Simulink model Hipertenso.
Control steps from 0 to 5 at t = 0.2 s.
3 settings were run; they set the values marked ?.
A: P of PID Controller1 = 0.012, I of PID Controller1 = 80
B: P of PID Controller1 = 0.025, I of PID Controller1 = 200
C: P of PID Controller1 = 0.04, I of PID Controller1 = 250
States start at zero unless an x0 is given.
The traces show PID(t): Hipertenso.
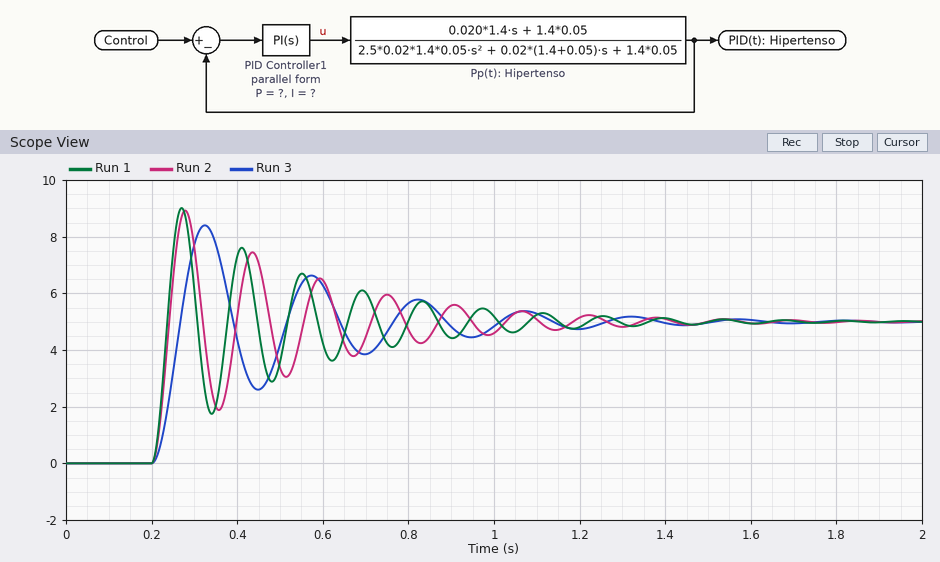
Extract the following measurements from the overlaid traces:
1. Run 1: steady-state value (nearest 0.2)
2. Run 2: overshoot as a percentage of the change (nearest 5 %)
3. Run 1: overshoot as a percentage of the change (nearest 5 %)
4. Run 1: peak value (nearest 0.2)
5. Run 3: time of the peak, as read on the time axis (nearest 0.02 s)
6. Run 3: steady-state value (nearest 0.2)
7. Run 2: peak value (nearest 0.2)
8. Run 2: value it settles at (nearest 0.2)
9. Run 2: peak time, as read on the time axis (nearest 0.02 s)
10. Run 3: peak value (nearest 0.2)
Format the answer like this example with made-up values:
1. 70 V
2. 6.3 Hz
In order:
1. 5.0
2. 80 %
3. 80 %
4. 9.0
5. 0.32 s
6. 5.0
7. 9.0
8. 5.0
9. 0.28 s
10. 8.4
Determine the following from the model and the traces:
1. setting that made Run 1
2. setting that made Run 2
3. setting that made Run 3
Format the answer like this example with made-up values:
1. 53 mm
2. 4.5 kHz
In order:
1. C
2. B
3. A
